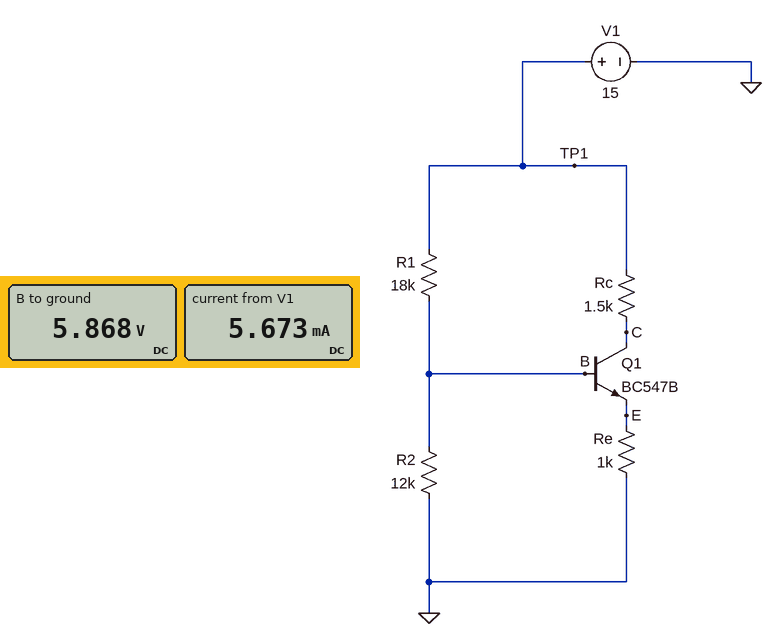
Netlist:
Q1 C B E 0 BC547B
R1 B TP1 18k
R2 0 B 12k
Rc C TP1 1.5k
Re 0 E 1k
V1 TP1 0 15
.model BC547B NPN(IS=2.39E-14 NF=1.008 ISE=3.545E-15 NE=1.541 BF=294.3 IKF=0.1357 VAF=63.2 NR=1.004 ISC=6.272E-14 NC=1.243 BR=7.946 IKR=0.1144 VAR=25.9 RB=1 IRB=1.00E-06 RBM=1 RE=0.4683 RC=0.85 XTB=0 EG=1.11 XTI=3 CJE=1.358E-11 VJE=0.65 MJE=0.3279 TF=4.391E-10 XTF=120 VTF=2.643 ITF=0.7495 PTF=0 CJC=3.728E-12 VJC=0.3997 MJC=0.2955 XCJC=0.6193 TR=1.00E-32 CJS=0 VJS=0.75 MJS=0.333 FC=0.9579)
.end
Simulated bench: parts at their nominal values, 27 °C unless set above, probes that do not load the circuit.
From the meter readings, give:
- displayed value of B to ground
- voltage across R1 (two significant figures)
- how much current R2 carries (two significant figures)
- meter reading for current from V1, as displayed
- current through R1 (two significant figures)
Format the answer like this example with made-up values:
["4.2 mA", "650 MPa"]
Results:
["5.868 V", "9.1 V", "490 µA", "5.673 mA", "510 µA"]
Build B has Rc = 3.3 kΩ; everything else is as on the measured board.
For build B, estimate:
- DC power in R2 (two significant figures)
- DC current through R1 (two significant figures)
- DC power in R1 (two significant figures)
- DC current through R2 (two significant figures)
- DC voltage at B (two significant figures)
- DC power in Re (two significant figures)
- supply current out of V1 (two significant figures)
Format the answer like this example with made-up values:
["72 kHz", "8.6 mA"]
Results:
["1.6 mW", "590 µA", "6.3 mW", "360 µA", "4.3 V", "13 mW", "4.0 mA"]
